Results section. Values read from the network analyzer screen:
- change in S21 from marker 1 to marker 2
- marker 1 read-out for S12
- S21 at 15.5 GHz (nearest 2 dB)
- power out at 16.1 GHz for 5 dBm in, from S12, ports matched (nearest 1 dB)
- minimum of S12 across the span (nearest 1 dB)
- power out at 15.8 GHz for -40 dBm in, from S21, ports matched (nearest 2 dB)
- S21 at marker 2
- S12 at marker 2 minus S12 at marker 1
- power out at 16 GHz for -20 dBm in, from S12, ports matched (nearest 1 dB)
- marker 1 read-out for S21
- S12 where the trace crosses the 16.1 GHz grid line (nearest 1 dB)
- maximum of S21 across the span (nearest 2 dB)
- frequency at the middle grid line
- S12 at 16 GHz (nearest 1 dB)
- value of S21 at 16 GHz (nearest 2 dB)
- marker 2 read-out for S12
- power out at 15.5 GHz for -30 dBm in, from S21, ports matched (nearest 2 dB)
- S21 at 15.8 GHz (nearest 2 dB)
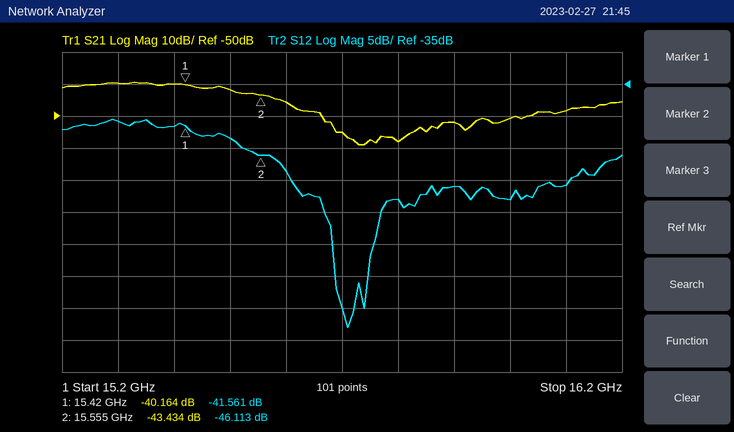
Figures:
-3.270 dB
-41.561 dB
-42 dB
-46 dBm
-73 dB
-98 dBm
-43.434 dB
-4.552 dB
-73 dBm
-40.164 dB
-51 dB
-40 dB
15.7 GHz
-53 dB
-50 dB
-46.113 dB
-72 dBm
-58 dB
